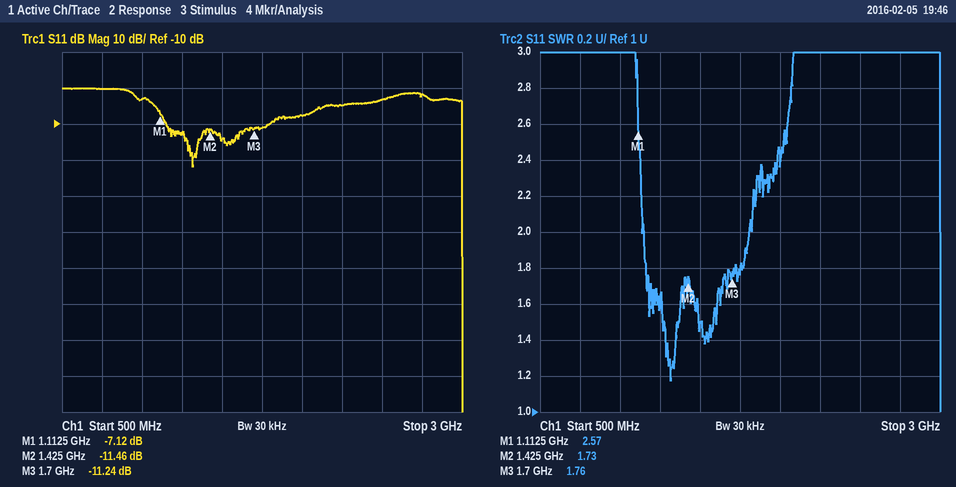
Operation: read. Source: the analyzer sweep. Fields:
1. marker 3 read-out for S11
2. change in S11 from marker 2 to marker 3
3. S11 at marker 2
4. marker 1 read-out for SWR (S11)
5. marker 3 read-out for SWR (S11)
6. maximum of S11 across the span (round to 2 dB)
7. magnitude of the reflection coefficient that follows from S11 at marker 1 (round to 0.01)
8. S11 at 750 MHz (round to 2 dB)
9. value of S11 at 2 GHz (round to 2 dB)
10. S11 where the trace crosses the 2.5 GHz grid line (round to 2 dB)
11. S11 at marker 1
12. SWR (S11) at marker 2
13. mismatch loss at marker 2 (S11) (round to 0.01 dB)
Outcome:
-11.24 dB
0.22 dB
-11.46 dB
2.57
1.76
0 dB
0.44
0 dB
-8 dB
-4 dB
-7.12 dB
1.73
0.32 dB
